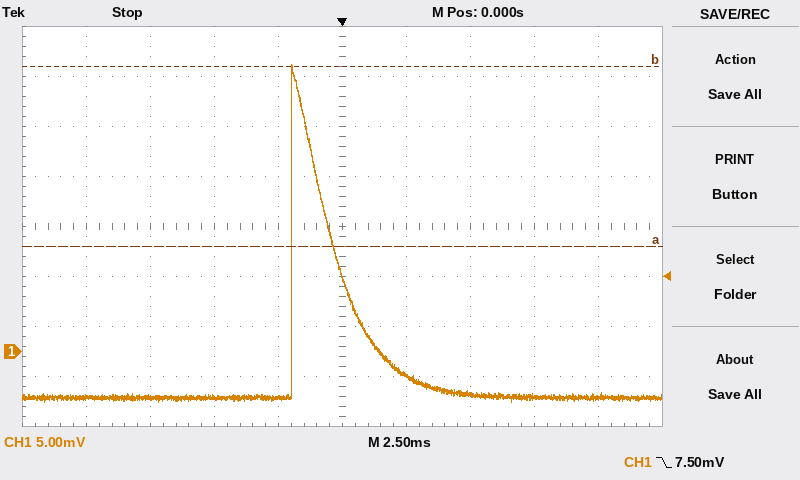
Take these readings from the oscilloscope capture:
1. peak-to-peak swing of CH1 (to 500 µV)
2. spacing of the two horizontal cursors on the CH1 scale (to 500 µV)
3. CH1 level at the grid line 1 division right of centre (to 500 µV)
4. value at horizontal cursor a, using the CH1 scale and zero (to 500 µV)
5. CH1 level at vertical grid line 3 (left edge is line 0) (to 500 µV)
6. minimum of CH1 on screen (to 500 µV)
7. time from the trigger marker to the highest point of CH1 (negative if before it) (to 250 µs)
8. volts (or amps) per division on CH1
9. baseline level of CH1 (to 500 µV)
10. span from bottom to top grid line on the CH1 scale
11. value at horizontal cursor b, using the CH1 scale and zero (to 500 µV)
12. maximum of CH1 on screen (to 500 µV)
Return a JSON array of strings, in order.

["33.5 mV", "18.0 mV", "-2.5 mV", "10.5 mV", "-4.5 mV", "-5.0 mV", "-2.00 ms", "5 mV", "-4.5 mV", "40 mV", "28.5 mV", "28.5 mV"]
